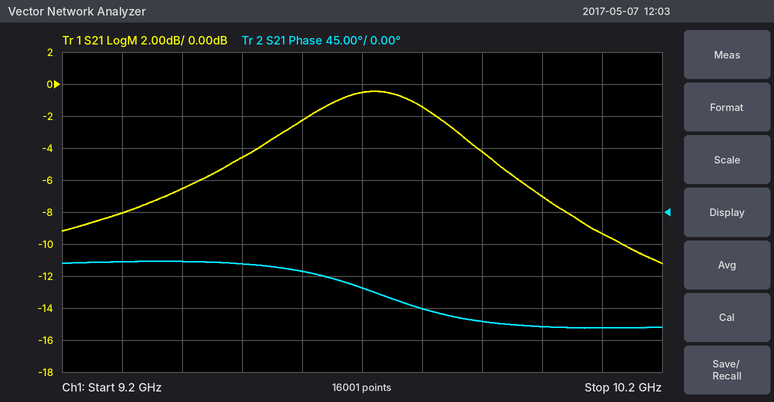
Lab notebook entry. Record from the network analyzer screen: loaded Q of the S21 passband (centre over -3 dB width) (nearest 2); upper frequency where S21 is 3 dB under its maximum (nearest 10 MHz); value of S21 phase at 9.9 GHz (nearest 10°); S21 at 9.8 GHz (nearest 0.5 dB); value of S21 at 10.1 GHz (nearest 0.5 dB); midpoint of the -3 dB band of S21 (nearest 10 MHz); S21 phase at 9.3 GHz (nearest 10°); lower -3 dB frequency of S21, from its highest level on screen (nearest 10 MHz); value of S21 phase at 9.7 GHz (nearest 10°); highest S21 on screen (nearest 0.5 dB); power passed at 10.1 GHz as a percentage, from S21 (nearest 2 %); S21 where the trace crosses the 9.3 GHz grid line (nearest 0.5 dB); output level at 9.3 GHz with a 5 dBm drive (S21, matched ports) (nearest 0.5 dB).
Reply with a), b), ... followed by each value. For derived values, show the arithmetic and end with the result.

a) 9.71 GHz / 320 MHz ≈ 30
b) 9.87 GHz
c) -150°
d) -1.5 dB
e) -9.5 dB
f) 9.71 GHz
g) -70°
h) 9.55 GHz
i) -110°
j) -0.5 dB
k) 10^(-9.5/10) ≈ 11.2 %, so 12 % to the nearest 2 %
l) -8.0 dB
m) 5 dBm + (-8.0 dB) = -3.0 dBm
